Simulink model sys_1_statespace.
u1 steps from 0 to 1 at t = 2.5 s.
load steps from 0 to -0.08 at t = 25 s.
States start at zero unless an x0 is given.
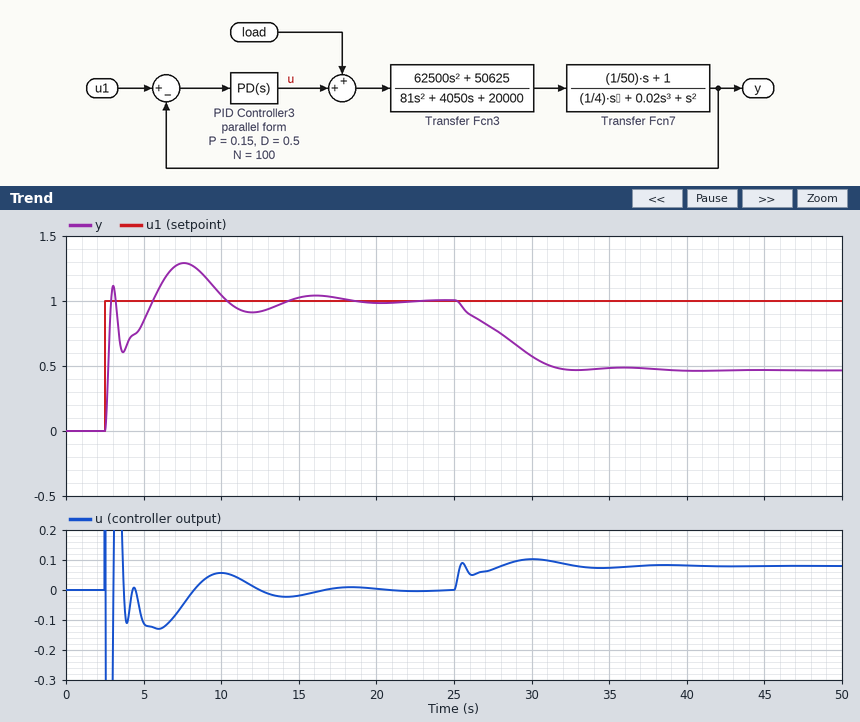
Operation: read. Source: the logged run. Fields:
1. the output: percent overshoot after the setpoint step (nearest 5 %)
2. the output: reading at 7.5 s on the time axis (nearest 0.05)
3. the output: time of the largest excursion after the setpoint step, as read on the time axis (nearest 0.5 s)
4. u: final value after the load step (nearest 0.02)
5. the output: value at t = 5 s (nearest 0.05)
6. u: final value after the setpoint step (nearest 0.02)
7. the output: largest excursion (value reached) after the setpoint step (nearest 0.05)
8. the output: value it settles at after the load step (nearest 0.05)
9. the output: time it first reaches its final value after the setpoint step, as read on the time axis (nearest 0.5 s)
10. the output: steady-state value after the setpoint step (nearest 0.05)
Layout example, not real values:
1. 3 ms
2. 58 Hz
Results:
1. 30 %
2. 1.30
3. 7.5 s
4. 0.08
5. 0.85
6. 0.00
7. 1.30
8. 0.45
9. 3.0 s
10. 1.00
